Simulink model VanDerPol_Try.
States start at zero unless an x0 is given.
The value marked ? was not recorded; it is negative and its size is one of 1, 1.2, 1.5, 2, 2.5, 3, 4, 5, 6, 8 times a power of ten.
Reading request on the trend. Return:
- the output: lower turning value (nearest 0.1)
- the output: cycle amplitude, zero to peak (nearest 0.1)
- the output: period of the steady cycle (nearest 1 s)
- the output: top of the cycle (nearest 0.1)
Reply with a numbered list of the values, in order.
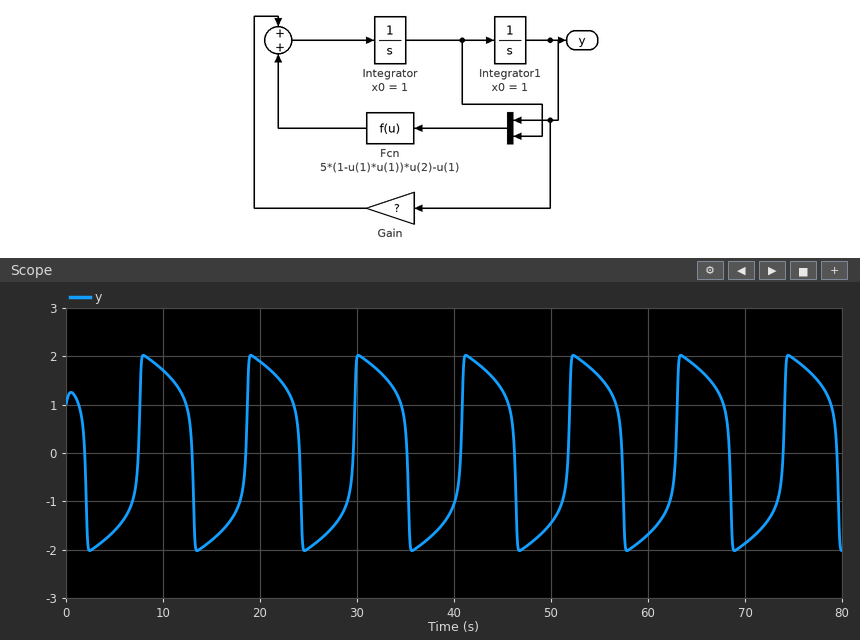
1. -2.0
2. 2.0
3. 11 s
4. 2.0
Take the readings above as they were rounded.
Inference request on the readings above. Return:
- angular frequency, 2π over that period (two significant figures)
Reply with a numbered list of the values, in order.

1. 0.57 rad/s
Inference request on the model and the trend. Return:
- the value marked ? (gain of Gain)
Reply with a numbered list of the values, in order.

1. -0.06
